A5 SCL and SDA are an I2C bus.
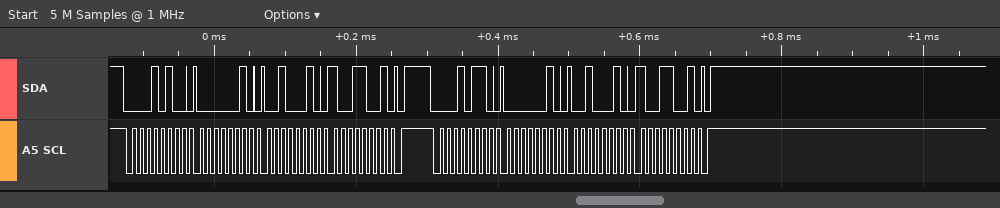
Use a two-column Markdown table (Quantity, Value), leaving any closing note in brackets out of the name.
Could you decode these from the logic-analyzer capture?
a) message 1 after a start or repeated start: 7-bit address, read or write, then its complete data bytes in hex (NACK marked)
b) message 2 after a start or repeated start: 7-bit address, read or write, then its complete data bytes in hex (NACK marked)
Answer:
| Quantity | Value |
|---|---|
| message 1 after a start or repeated start: 7-bit address, read or write, then its complete data bytes in hex | 0x0A write: 02 22 99 |
| message 2 after a start or repeated start: 7-bit address, read or write, then its complete data bytes in hex | 0x0B write: 02 22 99 |
